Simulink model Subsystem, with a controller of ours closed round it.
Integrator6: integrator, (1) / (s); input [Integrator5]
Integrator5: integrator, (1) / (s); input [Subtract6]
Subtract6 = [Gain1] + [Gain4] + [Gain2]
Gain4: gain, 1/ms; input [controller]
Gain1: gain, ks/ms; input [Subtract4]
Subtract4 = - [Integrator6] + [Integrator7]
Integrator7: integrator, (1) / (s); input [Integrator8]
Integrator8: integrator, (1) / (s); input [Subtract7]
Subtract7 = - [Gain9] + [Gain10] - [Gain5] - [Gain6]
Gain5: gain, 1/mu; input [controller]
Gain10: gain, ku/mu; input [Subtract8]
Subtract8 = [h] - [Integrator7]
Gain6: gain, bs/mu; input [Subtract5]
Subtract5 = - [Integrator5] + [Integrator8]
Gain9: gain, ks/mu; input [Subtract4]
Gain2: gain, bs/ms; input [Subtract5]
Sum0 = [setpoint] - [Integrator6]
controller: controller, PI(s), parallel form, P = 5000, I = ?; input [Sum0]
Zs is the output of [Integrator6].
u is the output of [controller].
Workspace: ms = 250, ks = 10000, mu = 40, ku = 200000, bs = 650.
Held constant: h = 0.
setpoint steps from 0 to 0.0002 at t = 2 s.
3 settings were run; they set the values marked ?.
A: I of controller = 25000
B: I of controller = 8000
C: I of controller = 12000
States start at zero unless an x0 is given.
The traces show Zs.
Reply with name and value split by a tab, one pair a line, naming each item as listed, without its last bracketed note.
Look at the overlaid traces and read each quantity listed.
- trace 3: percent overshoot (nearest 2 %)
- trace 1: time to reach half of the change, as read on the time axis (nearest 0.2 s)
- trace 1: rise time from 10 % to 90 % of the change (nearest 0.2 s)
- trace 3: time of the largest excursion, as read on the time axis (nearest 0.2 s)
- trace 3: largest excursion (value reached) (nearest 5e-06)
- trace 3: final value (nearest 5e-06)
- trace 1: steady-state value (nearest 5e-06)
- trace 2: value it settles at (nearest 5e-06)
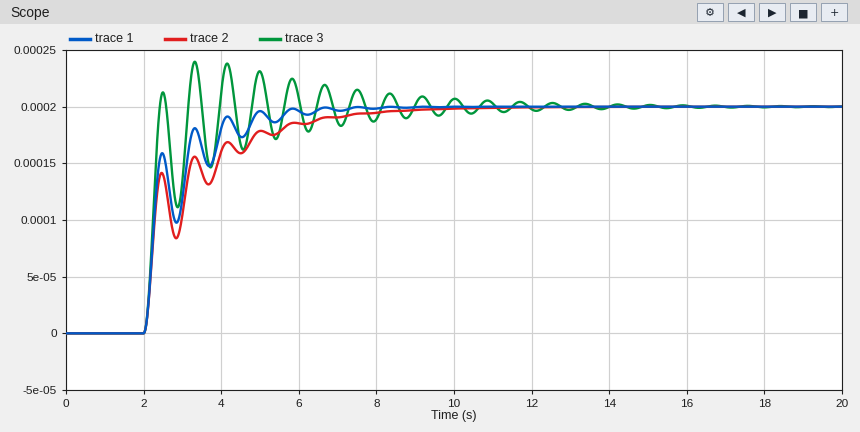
trace 3: percent overshoot	20 %
trace 1: time to reach half of the change, as read on the time axis	2.2 s
trace 1: rise time from 10 % to 90 % of the change	1.2 s
trace 3: time of the largest excursion, as read on the time axis	3.4 s
trace 3: largest excursion (value reached)	0.000240
trace 3: final value	0.000200
trace 1: steady-state value	0.000200
trace 2: value it settles at	0.000200
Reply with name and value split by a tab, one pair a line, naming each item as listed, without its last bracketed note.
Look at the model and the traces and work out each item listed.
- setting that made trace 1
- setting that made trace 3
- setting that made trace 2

setting that made trace 1	C
setting that made trace 3	A
setting that made trace 2	B
